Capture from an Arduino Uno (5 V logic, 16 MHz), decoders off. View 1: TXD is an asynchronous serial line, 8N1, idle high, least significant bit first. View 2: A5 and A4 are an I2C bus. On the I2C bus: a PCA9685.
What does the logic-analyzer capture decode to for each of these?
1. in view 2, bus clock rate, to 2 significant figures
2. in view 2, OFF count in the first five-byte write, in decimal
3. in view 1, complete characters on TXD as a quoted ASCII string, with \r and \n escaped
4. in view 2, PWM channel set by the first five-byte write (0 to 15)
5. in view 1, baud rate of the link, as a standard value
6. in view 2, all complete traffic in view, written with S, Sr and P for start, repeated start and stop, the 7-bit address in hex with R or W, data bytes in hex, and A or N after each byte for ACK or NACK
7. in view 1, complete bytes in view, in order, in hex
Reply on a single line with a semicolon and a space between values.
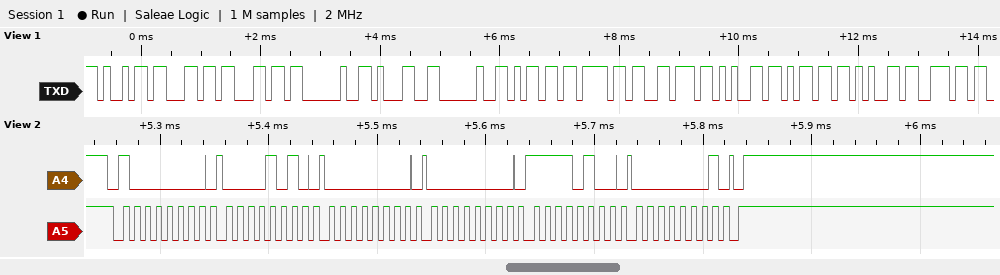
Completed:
100 kHz; 500; "ill 1 movemen"; 1; 9600 baud; S 40W A 0A A 00 A 00 A F4 A 01 A P; 0x69 0x6C 0x6C 0x20 0x31 0x20 0x6D 0x6F 0x76 0x65 0x6D 0x65 0x6E
